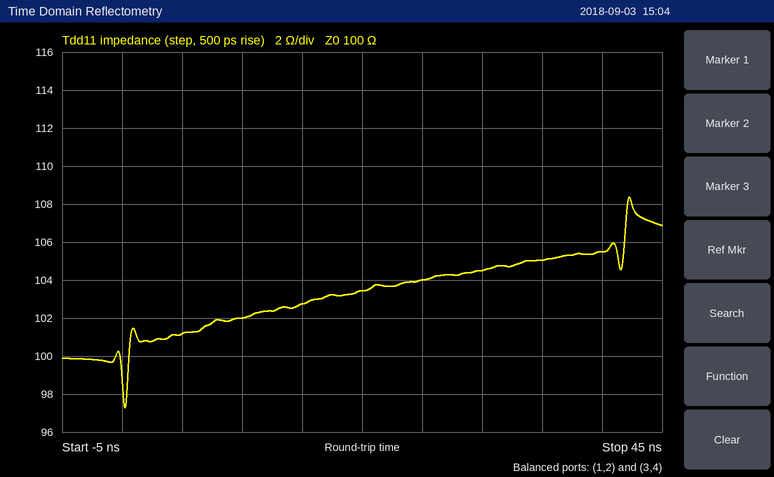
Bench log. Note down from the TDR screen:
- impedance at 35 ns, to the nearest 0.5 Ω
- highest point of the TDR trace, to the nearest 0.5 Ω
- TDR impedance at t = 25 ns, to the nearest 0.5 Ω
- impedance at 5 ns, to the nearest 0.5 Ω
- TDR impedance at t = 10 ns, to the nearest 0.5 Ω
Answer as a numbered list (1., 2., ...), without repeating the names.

1. 105.0 Ω
2. 108.5 Ω
3. 104.0 Ω
4. 101.0 Ω
5. 102.0 Ω
